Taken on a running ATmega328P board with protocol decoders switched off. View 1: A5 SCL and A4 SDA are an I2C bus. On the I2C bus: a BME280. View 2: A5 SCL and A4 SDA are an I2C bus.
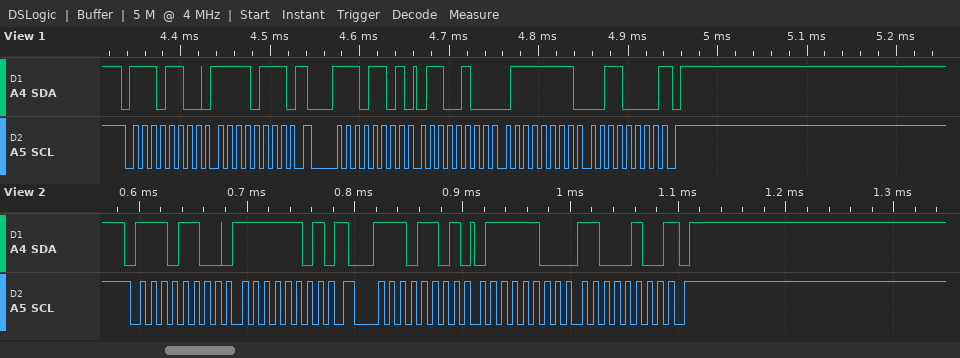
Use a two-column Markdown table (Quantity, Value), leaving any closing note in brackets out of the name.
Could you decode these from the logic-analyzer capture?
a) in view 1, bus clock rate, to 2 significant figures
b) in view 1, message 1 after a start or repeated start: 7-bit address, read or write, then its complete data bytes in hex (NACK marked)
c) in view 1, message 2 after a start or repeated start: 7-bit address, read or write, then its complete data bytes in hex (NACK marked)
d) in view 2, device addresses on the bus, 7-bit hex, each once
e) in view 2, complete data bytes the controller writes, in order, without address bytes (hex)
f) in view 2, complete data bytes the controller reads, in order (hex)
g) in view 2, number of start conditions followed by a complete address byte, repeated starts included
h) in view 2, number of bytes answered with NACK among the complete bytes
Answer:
| Quantity | Value |
|---|---|
| in view 1, bus clock rate, to 2 significant figures | 100 kHz |
| in view 1, message 1 after a start or repeated start: 7-bit address, read or write, then its complete data bytes in hex | 0x76 write: F7 |
| in view 1, message 2 after a start or repeated start: 7-bit address, read or write, then its complete data bytes in hex | 0x76 read: 64 7F 30 NACK |
| in view 2, device addresses on the bus, 7-bit hex, each once | 0x76 |
| in view 2, complete data bytes the controller writes, in order, without address bytes | FD |
| in view 2, complete data bytes the controller reads, in order | 7C C4 |
| in view 2, number of start conditions followed by a complete address byte, repeated starts included | 2 |
| in view 2, number of bytes answered with NACK among the complete bytes | 1 |
